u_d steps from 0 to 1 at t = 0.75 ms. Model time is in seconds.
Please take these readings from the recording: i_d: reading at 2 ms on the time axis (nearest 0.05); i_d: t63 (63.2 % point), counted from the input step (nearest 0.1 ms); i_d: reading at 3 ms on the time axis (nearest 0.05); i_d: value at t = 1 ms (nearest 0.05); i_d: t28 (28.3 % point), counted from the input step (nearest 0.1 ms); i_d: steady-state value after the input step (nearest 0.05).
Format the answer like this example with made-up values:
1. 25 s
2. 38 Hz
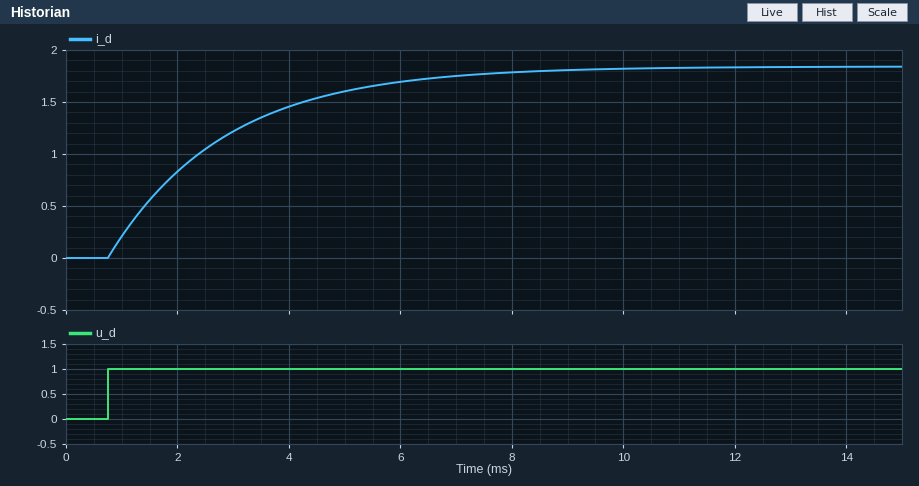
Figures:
1. 0.85
2. 2.1 ms
3. 1.20
4. 0.20
5. 0.7 ms
6. 1.85
